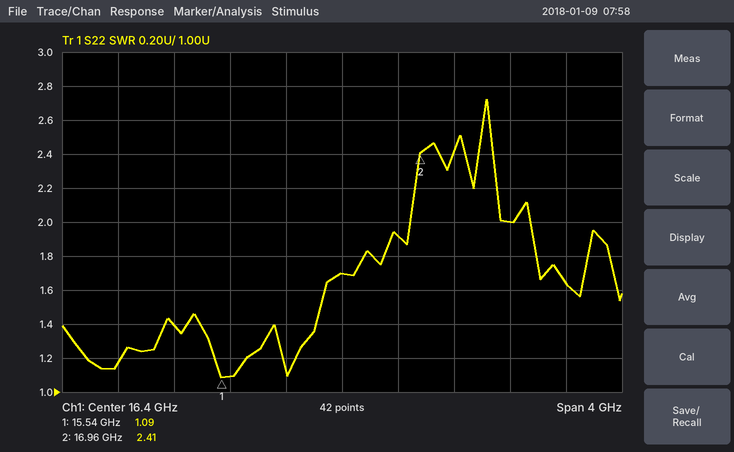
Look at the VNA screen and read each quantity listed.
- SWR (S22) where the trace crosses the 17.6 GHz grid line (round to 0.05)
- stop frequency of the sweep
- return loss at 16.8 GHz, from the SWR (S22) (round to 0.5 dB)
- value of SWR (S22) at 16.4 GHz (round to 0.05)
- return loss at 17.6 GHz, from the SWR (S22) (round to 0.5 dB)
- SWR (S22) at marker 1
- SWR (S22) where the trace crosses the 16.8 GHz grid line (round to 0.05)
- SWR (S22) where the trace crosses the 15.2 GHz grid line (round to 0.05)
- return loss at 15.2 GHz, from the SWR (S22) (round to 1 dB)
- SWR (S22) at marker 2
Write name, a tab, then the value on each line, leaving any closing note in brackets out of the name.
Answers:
SWR (S22) where the trace crosses the 17.6 GHz grid line	2.00
stop frequency of the sweep	18.4 GHz
return loss at 16.8 GHz, from the SWR (S22)	10.0 dB
value of SWR (S22) at 16.4 GHz	1.70
return loss at 17.6 GHz, from the SWR (S22)	9.5 dB
SWR (S22) at marker 1	1.09
SWR (S22) where the trace crosses the 16.8 GHz grid line	1.90
SWR (S22) where the trace crosses the 15.2 GHz grid line	1.40
return loss at 15.2 GHz, from the SWR (S22)	16 dB
SWR (S22) at marker 2	2.41
